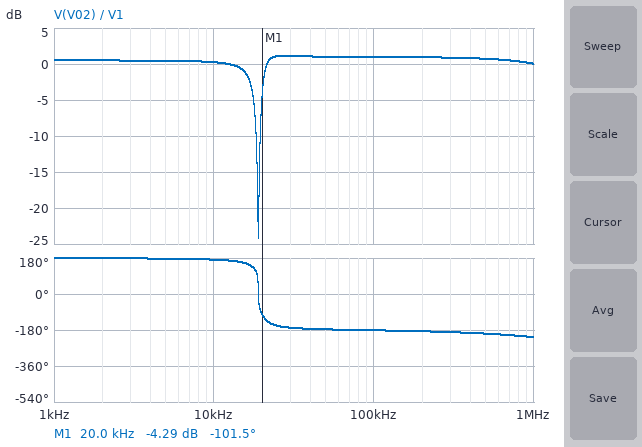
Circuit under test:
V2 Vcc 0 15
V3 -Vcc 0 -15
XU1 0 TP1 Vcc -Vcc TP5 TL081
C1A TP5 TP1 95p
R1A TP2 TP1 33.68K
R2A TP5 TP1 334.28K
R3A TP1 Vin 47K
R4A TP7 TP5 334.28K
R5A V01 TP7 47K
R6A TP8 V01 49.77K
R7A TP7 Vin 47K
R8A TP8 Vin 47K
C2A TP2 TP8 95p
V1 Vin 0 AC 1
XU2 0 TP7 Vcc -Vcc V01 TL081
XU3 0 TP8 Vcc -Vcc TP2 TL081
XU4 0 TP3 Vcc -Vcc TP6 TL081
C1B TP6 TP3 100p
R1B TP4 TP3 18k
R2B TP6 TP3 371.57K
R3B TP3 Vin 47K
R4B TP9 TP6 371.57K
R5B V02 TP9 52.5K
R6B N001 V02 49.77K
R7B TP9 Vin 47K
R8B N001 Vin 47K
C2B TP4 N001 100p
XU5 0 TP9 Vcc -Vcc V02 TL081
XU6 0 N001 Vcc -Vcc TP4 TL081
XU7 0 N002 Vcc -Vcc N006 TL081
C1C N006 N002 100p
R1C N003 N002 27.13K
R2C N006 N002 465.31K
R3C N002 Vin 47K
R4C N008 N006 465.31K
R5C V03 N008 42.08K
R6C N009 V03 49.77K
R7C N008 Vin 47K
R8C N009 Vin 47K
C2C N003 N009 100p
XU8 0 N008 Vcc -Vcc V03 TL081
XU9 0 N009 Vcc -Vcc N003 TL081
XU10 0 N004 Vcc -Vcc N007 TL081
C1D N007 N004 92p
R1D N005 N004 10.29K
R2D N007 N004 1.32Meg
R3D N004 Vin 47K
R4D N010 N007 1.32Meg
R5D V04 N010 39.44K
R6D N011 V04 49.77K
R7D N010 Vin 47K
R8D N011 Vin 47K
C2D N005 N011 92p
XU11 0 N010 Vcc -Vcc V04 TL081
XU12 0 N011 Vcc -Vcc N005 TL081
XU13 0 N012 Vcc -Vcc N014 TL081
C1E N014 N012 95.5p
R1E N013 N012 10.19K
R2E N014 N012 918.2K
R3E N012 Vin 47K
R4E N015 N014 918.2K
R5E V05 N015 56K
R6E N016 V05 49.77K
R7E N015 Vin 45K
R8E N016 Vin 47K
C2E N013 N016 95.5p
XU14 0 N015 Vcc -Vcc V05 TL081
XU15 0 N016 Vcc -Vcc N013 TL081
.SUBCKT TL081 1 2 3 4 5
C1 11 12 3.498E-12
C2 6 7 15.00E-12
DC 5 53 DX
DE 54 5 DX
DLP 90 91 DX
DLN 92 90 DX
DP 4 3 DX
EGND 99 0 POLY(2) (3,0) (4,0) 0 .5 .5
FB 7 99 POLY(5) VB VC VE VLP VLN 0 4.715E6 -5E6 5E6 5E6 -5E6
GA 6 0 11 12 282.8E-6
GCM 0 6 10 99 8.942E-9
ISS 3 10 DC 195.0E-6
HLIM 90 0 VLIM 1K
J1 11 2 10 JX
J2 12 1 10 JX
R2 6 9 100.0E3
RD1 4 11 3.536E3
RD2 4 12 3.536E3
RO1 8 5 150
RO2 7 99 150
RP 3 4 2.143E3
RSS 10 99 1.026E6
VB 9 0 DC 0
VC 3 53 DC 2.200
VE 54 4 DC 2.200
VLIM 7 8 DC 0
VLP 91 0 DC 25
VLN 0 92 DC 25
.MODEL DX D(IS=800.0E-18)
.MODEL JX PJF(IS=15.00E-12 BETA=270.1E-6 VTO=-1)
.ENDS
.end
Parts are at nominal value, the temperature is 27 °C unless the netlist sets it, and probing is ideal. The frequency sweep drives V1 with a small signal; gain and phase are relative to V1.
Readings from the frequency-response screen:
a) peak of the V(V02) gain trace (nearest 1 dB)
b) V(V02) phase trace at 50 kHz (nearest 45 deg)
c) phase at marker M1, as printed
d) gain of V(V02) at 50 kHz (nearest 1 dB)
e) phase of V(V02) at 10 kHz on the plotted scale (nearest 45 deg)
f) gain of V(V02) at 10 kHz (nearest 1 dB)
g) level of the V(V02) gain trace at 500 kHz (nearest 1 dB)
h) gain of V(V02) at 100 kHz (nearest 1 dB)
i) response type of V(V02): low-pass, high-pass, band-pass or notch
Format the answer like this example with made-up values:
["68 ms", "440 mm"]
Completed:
["1 dB", "-180 deg", "-101.5 deg", "1 dB", "180 deg", "0 dB", "1 dB", "1 dB", "notch"]
